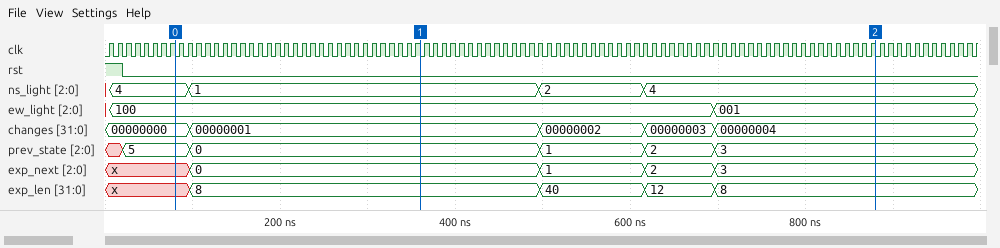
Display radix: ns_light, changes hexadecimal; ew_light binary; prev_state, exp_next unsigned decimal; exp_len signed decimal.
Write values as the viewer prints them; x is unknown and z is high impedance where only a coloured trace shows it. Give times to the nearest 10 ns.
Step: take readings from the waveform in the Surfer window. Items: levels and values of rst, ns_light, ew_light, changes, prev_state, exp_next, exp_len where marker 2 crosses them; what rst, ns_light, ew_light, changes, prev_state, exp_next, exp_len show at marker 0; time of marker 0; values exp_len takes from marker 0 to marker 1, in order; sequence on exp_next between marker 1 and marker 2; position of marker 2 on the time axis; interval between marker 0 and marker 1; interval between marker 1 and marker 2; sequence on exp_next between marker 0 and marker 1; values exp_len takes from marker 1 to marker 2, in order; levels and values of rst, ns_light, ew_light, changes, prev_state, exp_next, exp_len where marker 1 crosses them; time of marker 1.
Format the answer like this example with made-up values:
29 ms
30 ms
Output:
rst=0, ns_light=4, ew_light=001, changes=00000004, prev_state=3, exp_next=3, exp_len=8
rst=0, ns_light=4, ew_light=100, changes=00000000, prev_state=5, exp_next=x, exp_len=x
80 ns
x, 8
0, 1, 2, 3
880 ns
280 ns
520 ns
x, 0
8, 40, 12, 8
rst=0, ns_light=1, ew_light=100, changes=00000001, prev_state=0, exp_next=0, exp_len=8
360 ns
